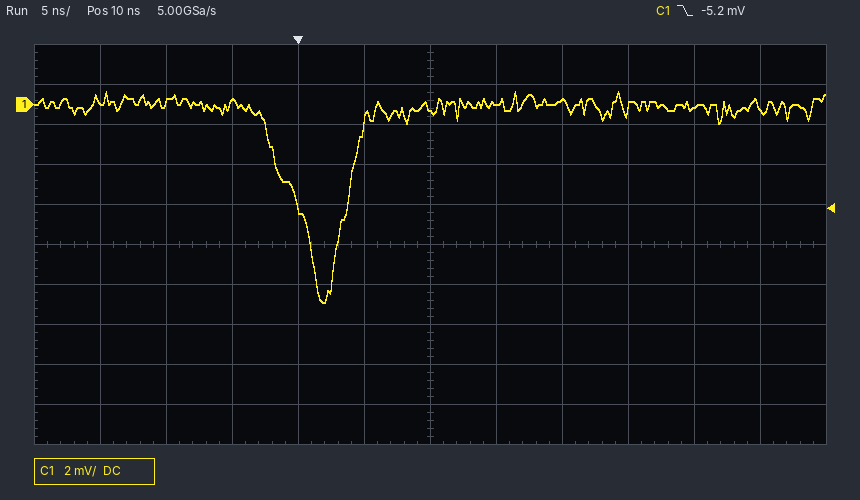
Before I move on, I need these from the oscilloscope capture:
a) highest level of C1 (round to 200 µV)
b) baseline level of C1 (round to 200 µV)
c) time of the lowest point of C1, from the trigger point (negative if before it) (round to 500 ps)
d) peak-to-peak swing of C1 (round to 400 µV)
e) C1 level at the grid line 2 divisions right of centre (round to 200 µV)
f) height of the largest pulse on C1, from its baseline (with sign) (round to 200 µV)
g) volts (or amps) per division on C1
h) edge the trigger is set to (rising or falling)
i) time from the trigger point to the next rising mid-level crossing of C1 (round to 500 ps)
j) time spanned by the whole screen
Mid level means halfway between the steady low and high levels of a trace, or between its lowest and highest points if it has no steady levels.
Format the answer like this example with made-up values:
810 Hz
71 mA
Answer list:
600 µV
0.0 mV
+2.0 ns
10.4 mV
200 µV
-9.8 mV
2 mV
falling
4.0 ns
60 ns
